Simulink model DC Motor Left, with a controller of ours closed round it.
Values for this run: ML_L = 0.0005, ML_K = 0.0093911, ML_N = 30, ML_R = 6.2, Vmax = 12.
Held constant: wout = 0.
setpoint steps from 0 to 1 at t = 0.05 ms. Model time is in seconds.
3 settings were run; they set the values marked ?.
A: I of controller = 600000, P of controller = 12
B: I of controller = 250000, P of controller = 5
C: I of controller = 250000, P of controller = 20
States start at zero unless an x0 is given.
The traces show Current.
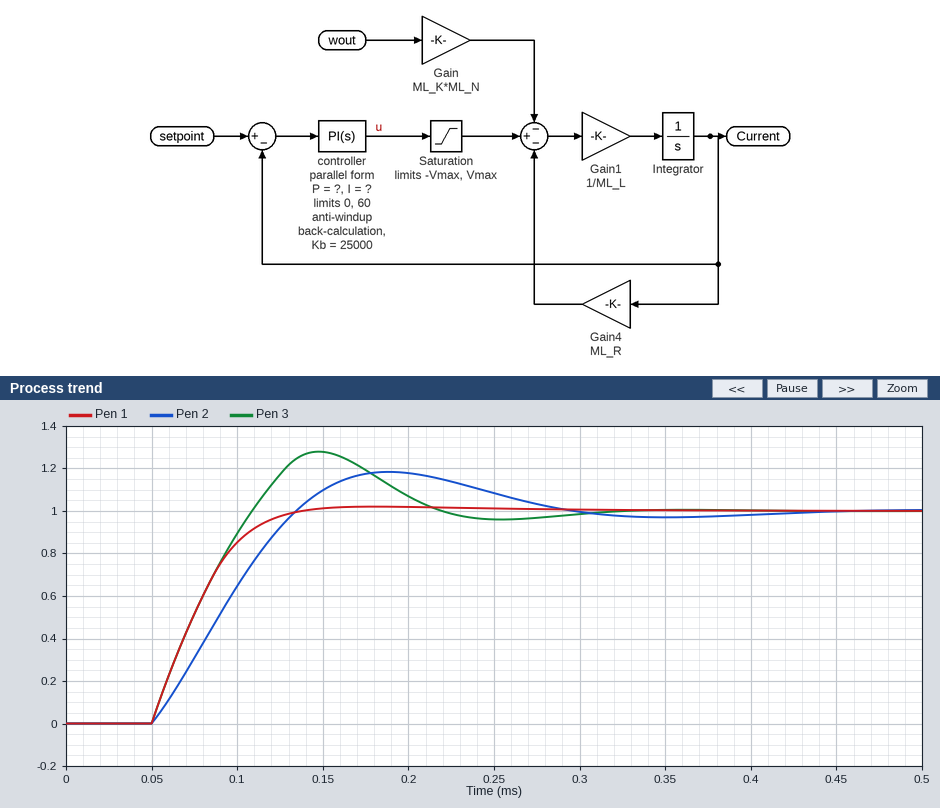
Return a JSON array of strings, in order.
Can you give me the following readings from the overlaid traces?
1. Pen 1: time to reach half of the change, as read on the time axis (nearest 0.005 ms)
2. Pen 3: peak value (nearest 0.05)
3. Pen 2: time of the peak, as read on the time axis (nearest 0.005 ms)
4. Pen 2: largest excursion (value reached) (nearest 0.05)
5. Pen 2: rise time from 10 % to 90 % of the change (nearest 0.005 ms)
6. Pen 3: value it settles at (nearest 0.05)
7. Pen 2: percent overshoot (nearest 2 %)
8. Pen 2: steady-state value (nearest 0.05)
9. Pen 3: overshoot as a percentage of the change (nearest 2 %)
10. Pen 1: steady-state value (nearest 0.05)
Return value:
["0.075 ms", "1.30", "0.190 ms", "1.20", "0.065 ms", "1.00", "18 %", "1.00", "28 %", "1.00"]
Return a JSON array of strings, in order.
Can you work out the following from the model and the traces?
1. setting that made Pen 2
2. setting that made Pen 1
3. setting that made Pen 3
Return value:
["B", "C", "A"]
